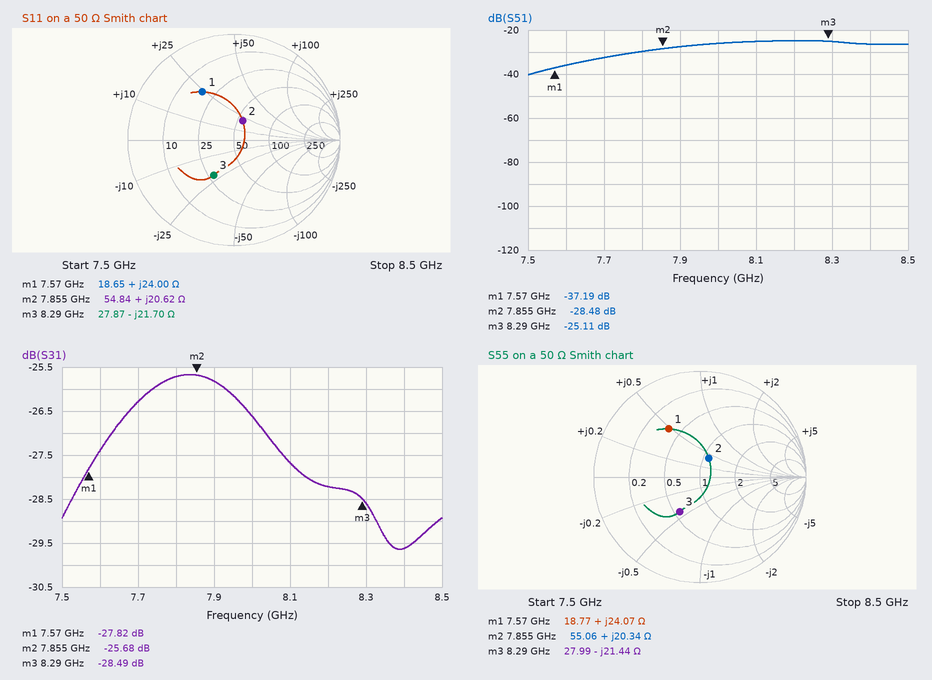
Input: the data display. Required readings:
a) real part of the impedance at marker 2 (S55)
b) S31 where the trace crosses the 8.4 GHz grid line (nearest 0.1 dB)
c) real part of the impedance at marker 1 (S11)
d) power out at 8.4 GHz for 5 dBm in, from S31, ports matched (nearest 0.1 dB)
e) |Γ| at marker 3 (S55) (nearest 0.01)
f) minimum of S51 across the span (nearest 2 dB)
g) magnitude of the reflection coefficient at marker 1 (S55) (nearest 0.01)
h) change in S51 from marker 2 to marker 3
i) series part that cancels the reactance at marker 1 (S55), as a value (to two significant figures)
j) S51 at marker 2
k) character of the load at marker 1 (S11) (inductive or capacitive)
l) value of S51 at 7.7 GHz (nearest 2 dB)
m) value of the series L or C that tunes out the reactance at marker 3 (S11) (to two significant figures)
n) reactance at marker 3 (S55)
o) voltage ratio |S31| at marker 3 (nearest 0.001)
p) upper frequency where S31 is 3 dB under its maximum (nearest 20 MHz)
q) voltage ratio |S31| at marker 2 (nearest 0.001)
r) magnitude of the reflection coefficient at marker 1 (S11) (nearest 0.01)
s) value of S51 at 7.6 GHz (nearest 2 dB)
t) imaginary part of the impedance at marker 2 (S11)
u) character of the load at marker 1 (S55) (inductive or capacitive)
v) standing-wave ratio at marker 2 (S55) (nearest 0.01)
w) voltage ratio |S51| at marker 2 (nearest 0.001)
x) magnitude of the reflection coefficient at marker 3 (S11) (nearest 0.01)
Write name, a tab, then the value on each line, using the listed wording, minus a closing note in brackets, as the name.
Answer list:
real part of the impedance at marker 2	55.06 Ω
S31 where the trace crosses the 8.4 GHz grid line	-29.6 dB
real part of the impedance at marker 1	18.65 Ω
power out at 8.4 GHz for 5 dBm in, from S31, ports matched	-24.6 dBm
|Γ| at marker 3 (S55)	0.38
minimum of S51 across the span	-40 dB
magnitude of the reflection coefficient at marker 1 (S55)	0.54
change in S51 from marker 2 to marker 3	3.37 dB
series part that cancels the reactance at marker 1 (S55), as a value	870 fF
S51 at marker 2	-28.48 dB
character of the load at marker 1 (S11)	inductive
value of S51 at 7.7 GHz	-32 dB
value of the series L or C that tunes out the reactance at marker 3 (S11)	420 pH
reactance at marker 3	-21.44 Ω
voltage ratio |S31| at marker 3	0.038
upper frequency where S31 is 3 dB under its maximum	8.30 GHz
voltage ratio |S31| at marker 2	0.052
magnitude of the reflection coefficient at marker 1 (S11)	0.54
value of S51 at 7.6 GHz	-36 dB
imaginary part of the impedance at marker 2	+20.62 Ω
character of the load at marker 1 (S55)	inductive
standing-wave ratio at marker 2 (S55)	1.49
voltage ratio |S51| at marker 2	0.038
magnitude of the reflection coefficient at marker 3 (S11)	0.38
